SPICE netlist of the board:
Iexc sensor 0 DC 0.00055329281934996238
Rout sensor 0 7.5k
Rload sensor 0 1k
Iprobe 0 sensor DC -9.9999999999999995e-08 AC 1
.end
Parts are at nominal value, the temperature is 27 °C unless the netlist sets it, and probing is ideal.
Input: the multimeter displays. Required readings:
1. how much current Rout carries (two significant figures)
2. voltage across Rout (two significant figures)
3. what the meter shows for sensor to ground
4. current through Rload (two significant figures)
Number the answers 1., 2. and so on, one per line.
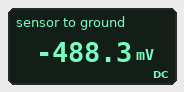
1. 65 µA
2. 490 mV
3. -488.3 mV
4. 490 µA
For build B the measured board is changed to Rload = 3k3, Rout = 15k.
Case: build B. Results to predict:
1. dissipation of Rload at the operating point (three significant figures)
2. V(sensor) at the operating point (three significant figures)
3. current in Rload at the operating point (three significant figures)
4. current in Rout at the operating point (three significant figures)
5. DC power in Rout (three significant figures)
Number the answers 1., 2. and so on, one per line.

1. 679 µW
2. -1.50 V
3. 454 µA
4. 99.8 µA
5. 149 µW
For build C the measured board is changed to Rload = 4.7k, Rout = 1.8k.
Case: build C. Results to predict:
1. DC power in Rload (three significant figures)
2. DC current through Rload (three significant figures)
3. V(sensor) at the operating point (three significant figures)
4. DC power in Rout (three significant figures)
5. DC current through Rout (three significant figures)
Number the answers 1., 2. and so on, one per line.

1. 110 µW
2. 153 µA
3. -720 mV
4. 288 µW
5. 400 µA
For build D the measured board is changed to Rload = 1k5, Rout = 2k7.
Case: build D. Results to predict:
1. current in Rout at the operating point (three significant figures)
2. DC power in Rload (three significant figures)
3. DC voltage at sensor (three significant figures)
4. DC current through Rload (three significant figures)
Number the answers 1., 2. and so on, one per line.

1. 198 µA
2. 190 µW
3. -534 mV
4. 356 µA
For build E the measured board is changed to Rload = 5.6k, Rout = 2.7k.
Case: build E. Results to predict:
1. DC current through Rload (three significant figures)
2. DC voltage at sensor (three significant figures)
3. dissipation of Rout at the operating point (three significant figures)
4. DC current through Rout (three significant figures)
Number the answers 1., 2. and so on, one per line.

1. 180 µA
2. -1.01 V
3. 376 µW
4. 373 µA
